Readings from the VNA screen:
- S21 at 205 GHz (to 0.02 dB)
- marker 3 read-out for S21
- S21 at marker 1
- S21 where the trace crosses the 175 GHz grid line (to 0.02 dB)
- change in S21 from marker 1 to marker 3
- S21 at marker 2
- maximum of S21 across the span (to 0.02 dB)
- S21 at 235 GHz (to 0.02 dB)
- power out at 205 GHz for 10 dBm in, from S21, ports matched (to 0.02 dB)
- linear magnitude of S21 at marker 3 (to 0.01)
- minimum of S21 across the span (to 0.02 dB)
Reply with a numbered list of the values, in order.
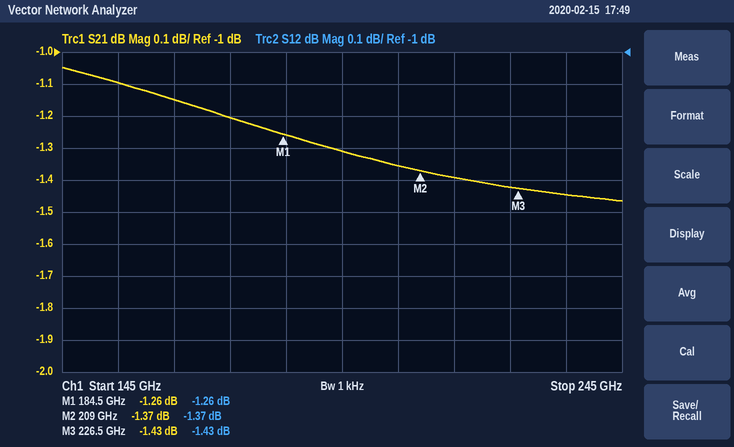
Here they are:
1. -1.36 dB
2. -1.43 dB
3. -1.26 dB
4. -1.20 dB
5. -0.17 dB
6. -1.37 dB
7. -1.04 dB
8. -1.44 dB
9. 8.64 dBm
10. 0.85
11. -1.46 dB
